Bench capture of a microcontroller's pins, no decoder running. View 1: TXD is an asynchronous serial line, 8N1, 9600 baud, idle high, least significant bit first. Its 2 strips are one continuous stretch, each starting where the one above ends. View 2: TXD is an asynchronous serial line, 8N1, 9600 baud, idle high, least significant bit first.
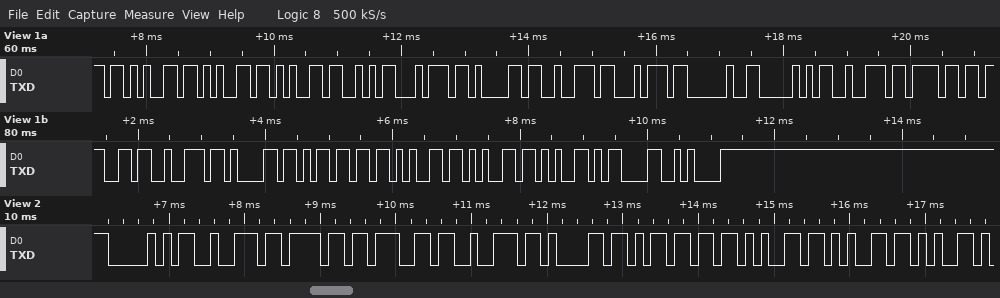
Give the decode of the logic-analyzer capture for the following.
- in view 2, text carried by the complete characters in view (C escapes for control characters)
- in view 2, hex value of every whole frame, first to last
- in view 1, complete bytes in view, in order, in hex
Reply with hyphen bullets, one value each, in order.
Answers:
- "Program+++"
- 50 72 6F 67 72 61 6D 2B 2B 2B
- 0x2B 0x2B 0x2B 0x53 0x74 0x61 0x72 0x74 0x20 0x50 0x72 0x6F 0x67 0x72 0x61 0x6D 0x2B 0x2B 0x2B 0x0D 0x0A
